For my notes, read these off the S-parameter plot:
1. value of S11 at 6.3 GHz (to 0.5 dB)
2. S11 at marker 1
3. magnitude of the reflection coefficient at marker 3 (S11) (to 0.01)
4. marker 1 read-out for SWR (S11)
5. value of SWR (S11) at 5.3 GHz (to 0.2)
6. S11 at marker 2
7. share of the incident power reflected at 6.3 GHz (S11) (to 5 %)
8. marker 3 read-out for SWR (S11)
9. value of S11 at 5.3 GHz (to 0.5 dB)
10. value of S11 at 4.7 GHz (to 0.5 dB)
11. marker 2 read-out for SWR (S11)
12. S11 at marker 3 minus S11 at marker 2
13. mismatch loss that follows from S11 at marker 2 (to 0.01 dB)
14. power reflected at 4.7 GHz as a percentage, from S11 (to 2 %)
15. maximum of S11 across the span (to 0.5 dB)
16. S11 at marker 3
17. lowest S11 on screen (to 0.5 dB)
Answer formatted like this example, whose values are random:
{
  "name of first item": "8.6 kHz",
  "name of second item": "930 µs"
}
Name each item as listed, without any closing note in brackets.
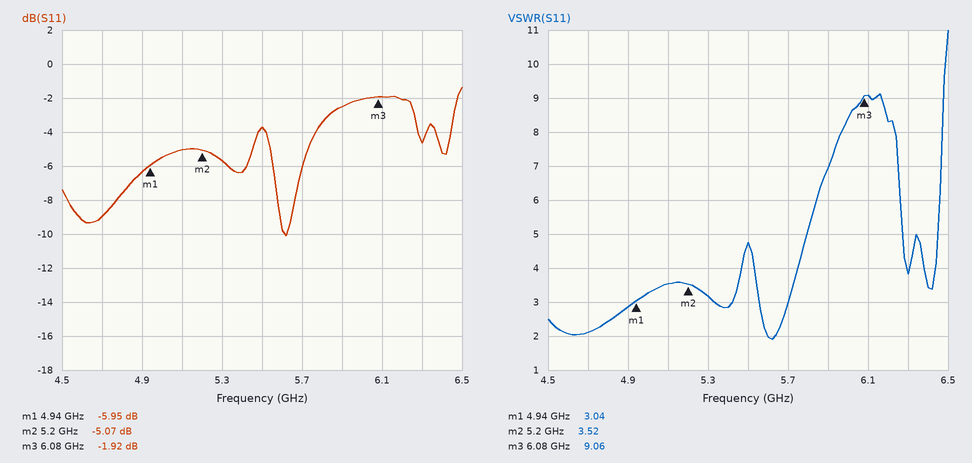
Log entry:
{
  "value of S11 at 6.3 GHz": "-4.5 dB",
  "S11 at marker 1": "-5.95 dB",
  "magnitude of the reflection coefficient at marker 3 (S11)": "0.80",
  "marker 1 read-out for SWR": "3.04",
  "value of SWR (S11) at 5.3 GHz": "3.2",
  "S11 at marker 2": "-5.07 dB",
  "share of the incident power reflected at 6.3 GHz (S11)": "35 %",
  "marker 3 read-out for SWR": "9.06",
  "value of S11 at 5.3 GHz": "-5.5 dB",
  "value of S11 at 4.7 GHz": "-9.0 dB",
  "marker 2 read-out for SWR": "3.52",
  "S11 at marker 3 minus S11 at marker 2": "3.15 dB",
  "mismatch loss that follows from S11 at marker 2": "1.62 dB",
  "power reflected at 4.7 GHz as a percentage, from S11": "12 %",
  "maximum of S11 across the span": "-1.5 dB",
  "S11 at marker 3": "-1.92 dB",
  "lowest S11 on screen": "-10.0 dB"
}
